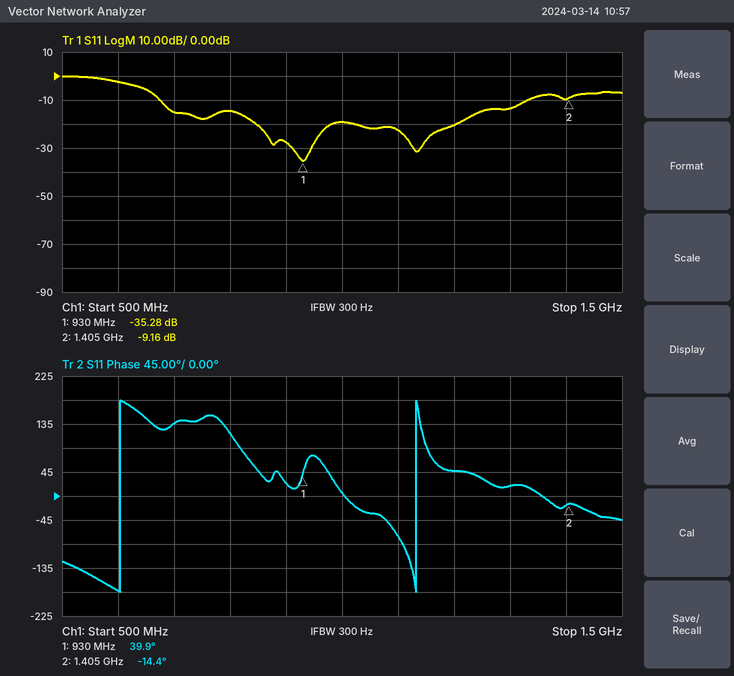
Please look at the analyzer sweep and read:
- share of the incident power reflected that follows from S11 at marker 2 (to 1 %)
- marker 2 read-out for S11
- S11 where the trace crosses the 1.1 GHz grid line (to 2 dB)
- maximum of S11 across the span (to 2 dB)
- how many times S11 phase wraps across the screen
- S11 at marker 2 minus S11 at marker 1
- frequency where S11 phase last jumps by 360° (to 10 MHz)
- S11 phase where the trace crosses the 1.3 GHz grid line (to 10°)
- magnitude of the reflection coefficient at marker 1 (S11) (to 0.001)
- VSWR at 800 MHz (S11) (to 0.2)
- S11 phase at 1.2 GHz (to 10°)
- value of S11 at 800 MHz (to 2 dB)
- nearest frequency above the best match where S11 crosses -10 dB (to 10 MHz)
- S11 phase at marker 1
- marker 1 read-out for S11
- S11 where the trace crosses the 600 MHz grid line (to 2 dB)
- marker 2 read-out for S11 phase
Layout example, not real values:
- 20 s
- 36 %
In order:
- 12 %
- -9.16 dB
- -22 dB
- 0 dB
- 2
- 26.12 dB
- 1.13 GHz
- 20°
- 0.017
- 1.4
- 50°
- -14 dB
- 1.33 GHz
- 39.9°
- -35.28 dB
- -2 dB
- -14.4°
